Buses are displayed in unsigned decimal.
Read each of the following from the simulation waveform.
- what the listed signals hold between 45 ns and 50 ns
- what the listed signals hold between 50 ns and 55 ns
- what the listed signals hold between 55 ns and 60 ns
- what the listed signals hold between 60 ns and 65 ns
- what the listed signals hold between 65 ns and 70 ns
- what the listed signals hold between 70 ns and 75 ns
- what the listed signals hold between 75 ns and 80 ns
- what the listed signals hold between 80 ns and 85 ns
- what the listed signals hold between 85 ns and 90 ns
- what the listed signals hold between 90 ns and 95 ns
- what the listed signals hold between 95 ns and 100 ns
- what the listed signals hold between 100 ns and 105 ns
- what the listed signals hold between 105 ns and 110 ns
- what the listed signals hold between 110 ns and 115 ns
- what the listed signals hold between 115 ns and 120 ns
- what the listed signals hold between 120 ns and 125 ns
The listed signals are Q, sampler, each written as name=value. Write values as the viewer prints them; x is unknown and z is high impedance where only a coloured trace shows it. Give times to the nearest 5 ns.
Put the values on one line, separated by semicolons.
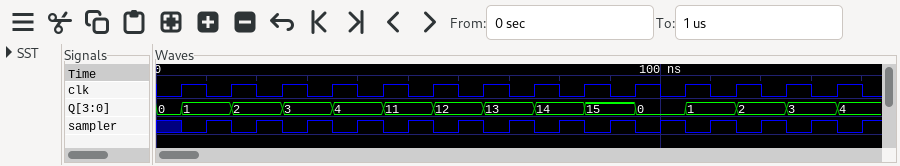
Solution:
Q=11, sampler=0; Q=11, sampler=1; Q=12, sampler=0; Q=12, sampler=1; Q=13, sampler=0; Q=13, sampler=1; Q=14, sampler=0; Q=14, sampler=1; Q=15, sampler=0; Q=15, sampler=1; Q=0, sampler=0; Q=0, sampler=1; Q=1, sampler=0; Q=1, sampler=1; Q=2, sampler=0; Q=2, sampler=1
